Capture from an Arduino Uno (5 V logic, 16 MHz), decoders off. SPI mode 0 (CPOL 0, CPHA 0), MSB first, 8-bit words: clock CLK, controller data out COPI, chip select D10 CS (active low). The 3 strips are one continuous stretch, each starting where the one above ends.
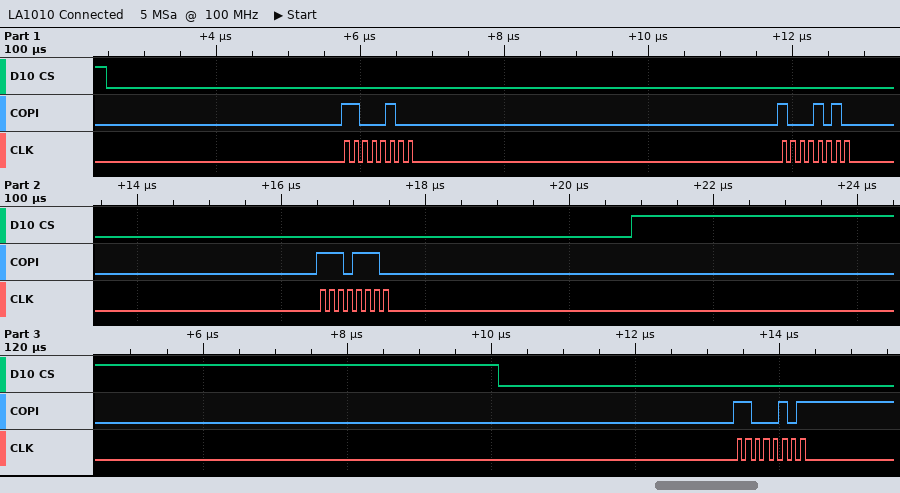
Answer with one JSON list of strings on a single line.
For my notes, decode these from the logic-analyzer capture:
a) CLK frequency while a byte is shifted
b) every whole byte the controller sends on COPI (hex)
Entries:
["8 MHz", "0xC4 0x8A 0xEE 0xC5"]
